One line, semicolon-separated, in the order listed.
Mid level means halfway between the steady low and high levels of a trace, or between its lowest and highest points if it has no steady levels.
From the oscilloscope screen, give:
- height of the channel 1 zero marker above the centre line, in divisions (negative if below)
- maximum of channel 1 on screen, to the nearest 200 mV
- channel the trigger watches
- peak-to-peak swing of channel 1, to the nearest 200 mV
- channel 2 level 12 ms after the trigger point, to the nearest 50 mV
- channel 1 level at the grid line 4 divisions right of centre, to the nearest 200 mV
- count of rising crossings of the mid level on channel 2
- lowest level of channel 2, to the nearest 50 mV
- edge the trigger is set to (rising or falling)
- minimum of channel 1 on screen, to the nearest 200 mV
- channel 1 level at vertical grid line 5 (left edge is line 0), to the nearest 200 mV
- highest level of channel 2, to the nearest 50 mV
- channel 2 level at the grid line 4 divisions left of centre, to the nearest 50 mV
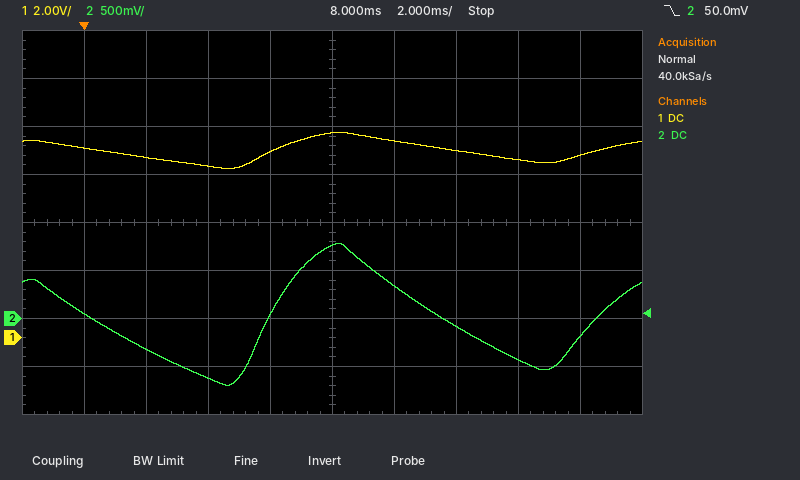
-2.4 div; 8.6 V; channel 2; 1.6 V; -100 mV; 7.6 V; 2; -700 mV; falling; 7.0 V; 8.6 V; 800 mV; 50 mV
